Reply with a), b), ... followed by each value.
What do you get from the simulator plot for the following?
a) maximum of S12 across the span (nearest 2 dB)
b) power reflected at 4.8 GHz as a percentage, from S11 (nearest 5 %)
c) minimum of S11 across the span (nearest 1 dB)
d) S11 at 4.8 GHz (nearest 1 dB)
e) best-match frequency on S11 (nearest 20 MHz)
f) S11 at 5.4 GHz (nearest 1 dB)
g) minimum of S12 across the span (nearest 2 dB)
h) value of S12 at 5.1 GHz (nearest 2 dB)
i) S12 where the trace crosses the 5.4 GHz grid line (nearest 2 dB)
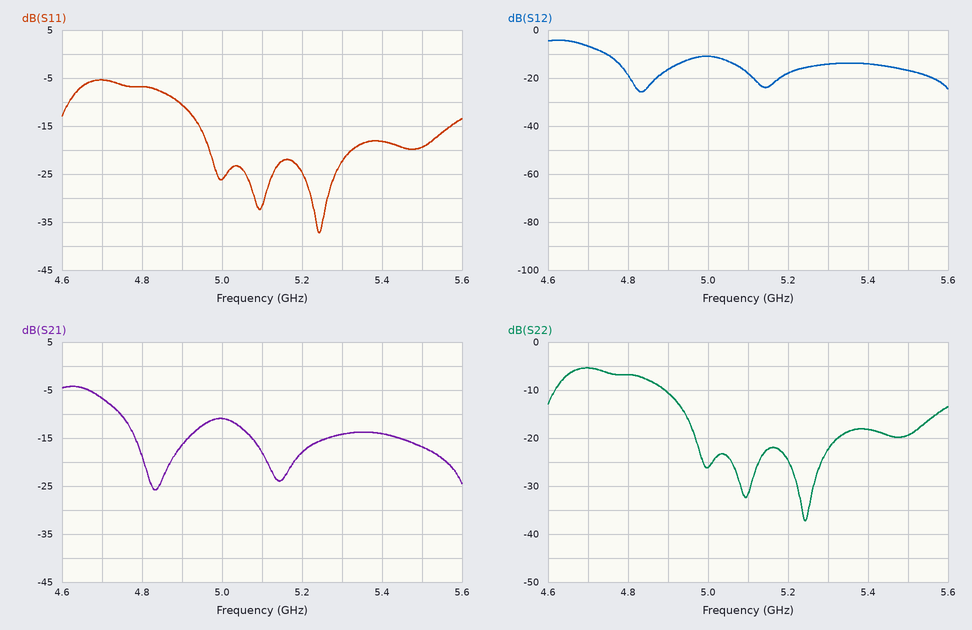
a) -4 dB
b) 20 %
c) -37 dB
d) -7 dB
e) 5.24 GHz
f) -18 dB
g) -26 dB
h) -18 dB
i) -14 dB
